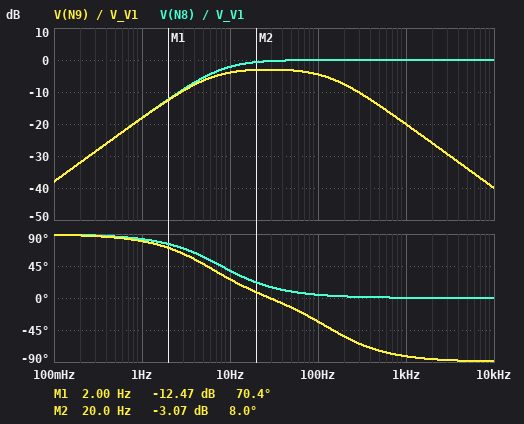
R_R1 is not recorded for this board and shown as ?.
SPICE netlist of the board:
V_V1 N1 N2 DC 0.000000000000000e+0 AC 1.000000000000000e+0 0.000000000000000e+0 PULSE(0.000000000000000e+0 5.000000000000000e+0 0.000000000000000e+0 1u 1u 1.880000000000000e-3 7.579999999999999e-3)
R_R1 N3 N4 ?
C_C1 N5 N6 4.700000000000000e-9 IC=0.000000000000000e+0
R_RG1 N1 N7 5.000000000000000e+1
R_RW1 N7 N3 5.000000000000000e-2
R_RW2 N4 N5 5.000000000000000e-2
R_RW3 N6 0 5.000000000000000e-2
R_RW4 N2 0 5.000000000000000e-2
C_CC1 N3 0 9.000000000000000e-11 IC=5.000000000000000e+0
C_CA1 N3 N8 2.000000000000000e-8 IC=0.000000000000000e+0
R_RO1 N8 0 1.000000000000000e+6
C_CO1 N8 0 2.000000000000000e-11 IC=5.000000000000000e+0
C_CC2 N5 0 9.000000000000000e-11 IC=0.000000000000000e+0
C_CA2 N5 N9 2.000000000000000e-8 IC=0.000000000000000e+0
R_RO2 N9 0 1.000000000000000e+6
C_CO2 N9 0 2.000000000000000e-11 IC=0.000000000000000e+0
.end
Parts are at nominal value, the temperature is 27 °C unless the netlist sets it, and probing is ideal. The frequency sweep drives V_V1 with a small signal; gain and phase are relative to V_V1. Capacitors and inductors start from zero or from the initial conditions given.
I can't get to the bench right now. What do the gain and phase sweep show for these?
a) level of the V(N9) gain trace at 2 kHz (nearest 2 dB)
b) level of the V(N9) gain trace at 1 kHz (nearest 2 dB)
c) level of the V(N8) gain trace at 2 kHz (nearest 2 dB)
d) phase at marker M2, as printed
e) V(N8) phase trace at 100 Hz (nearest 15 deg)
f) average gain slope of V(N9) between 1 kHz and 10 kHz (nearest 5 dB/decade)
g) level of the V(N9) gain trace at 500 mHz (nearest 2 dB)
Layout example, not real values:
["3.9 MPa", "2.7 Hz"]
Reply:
["-26 dB", "-20 dB", "0 dB", "8.0 deg", "0 deg", "-20 dB/decade", "-24 dB"]
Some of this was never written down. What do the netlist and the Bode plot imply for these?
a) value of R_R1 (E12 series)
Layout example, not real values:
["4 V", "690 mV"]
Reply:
["330 kΩ"]
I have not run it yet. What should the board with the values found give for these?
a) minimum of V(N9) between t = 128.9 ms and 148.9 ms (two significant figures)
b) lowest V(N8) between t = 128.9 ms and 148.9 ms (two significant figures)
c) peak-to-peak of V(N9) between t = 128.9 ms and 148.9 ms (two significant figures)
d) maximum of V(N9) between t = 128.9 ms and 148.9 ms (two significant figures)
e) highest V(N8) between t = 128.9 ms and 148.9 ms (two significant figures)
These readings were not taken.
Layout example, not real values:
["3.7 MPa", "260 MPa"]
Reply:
["-840 mV", "-1.4 V", "2.9 V", "2.0 V", "3.9 V"]
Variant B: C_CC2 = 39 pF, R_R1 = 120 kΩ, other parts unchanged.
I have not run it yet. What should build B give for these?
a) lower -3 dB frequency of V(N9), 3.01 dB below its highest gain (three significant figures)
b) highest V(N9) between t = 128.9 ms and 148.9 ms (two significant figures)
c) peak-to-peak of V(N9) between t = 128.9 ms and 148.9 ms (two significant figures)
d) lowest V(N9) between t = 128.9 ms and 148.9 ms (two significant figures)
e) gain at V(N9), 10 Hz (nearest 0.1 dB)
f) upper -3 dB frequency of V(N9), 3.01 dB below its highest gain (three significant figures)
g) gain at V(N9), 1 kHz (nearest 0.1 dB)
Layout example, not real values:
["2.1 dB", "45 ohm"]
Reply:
["6.78 Hz", "3.2 V", "4.3 V", "-1.1 V", "-2.8 dB", "327 Hz", "-11.5 dB"]
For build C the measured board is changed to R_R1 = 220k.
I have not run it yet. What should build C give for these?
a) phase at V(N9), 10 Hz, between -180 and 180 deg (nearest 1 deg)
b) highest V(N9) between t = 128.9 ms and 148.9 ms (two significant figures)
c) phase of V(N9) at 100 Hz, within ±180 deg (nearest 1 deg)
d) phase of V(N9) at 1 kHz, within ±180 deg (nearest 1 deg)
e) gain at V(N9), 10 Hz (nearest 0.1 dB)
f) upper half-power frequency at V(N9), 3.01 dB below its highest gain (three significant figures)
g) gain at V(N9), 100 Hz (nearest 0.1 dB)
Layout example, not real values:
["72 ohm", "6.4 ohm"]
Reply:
["30 deg", "2.6 V", "-25 deg", "-79 deg", "-3.3 dB", "197 Hz", "-2.9 dB"]
